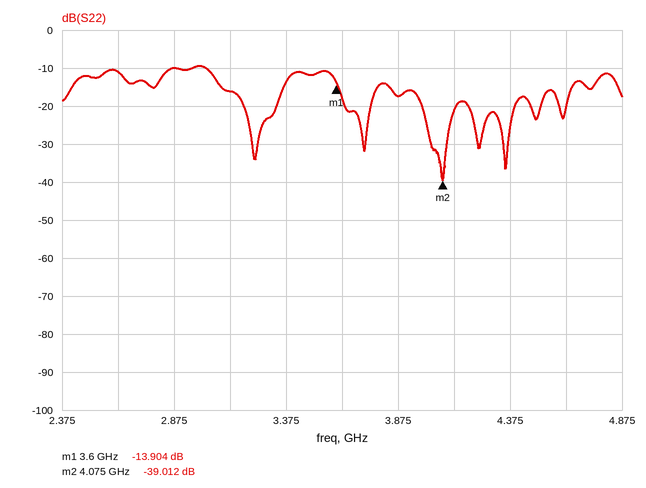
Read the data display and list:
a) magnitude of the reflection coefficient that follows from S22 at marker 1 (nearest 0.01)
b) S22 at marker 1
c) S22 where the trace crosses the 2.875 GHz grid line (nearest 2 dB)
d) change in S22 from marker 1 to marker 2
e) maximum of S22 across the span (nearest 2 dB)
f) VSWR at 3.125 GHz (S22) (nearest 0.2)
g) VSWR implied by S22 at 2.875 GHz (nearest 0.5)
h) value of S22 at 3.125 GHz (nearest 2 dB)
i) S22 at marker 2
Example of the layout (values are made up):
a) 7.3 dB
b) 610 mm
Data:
a) 0.20
b) -13.904 dB
c) -10 dB
d) -25.108 dB
e) -10 dB
f) 1.4
g) 2.0
h) -16 dB
i) -39.012 dB
